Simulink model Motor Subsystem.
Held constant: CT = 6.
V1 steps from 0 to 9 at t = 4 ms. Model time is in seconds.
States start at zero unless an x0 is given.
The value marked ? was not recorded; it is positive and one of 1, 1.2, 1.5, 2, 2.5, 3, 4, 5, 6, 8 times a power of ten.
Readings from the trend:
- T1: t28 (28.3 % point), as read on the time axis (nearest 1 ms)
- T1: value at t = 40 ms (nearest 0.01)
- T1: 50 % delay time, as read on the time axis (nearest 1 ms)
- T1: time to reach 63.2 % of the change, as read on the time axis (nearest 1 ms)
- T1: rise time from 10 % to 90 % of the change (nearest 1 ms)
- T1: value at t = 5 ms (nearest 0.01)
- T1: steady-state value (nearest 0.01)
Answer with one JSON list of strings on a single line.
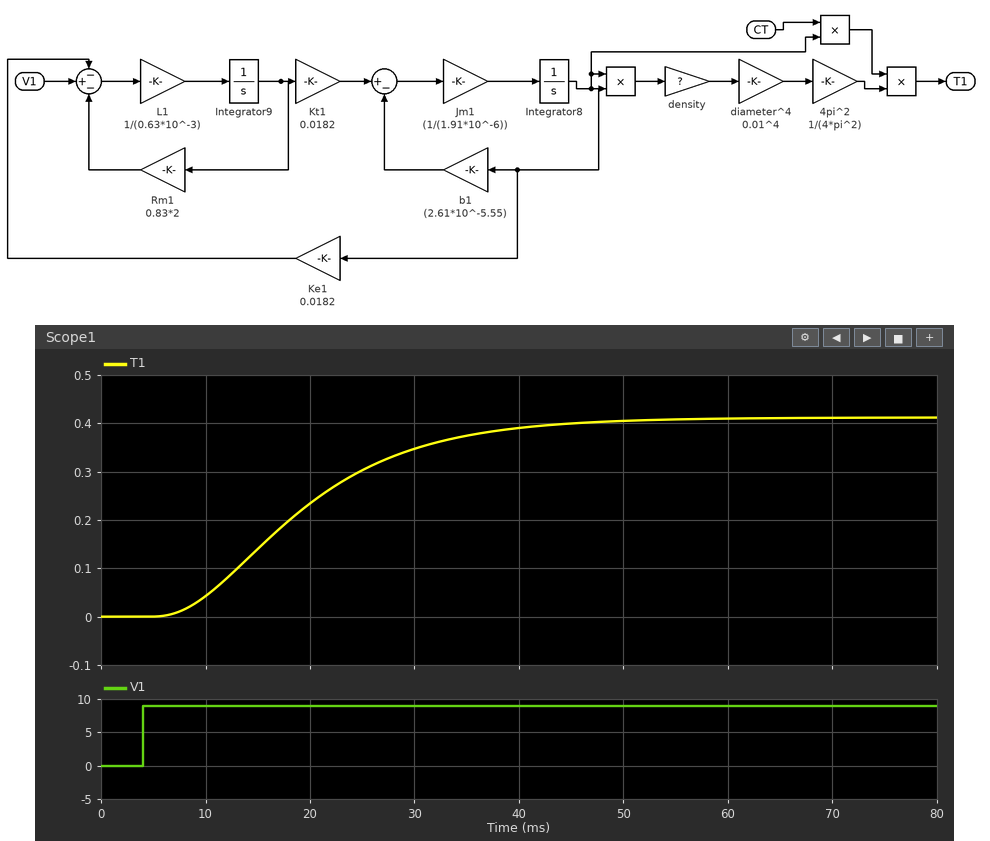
["14 ms", "0.39", "18 ms", "22 ms", "24 ms", "0.00", "0.41"]
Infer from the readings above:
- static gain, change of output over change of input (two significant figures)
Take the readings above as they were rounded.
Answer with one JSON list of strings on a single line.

["0.046"]
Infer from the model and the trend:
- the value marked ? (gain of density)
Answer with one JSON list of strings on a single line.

["2.5"]
